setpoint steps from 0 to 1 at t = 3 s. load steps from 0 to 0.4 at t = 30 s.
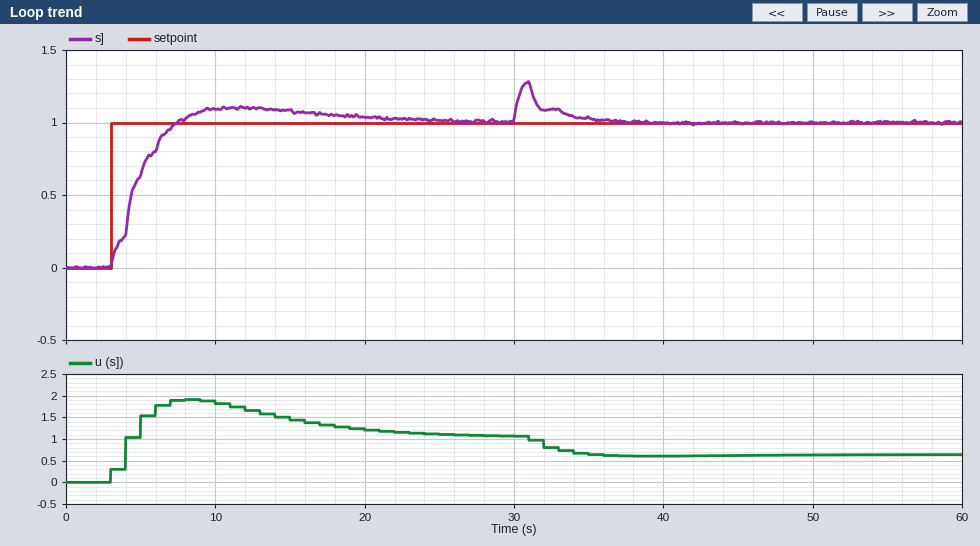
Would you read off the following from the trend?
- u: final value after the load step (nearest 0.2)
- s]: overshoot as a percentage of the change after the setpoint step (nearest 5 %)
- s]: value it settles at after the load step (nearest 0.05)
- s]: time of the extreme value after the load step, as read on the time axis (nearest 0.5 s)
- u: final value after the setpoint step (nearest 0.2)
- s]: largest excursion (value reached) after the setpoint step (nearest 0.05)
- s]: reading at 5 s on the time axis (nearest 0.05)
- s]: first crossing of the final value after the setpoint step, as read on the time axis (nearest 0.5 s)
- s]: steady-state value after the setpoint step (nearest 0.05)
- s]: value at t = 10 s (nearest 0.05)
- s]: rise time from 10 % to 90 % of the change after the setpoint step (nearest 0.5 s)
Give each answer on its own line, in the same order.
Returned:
0.6
10 %
1.00
31.0 s
1.0
1.10
0.65
7.5 s
1.00
1.10
3.0 s
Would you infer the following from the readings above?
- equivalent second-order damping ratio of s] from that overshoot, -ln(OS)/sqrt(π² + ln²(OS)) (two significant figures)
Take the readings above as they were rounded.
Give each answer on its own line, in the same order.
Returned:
0.59
